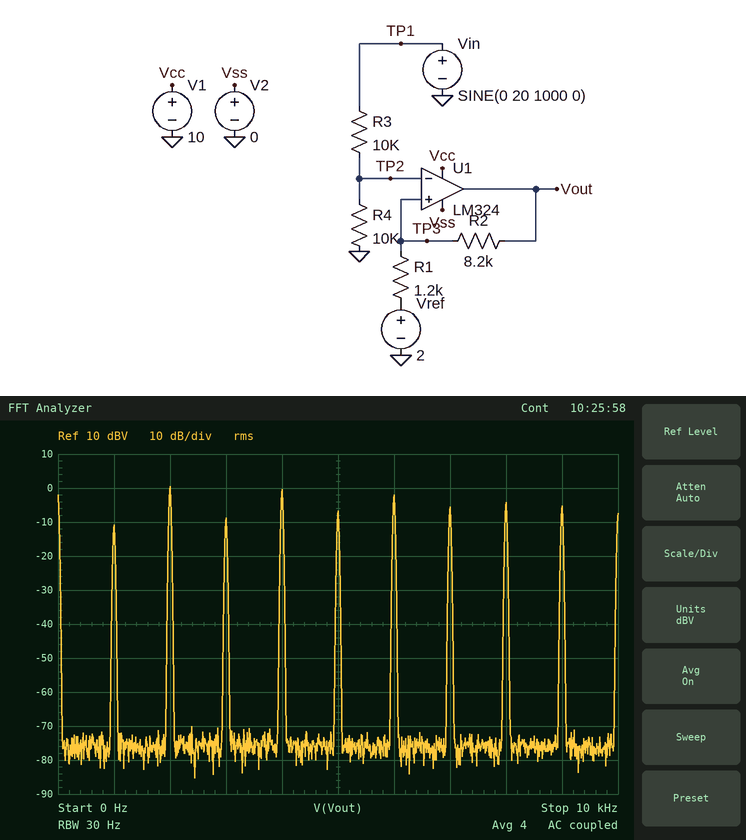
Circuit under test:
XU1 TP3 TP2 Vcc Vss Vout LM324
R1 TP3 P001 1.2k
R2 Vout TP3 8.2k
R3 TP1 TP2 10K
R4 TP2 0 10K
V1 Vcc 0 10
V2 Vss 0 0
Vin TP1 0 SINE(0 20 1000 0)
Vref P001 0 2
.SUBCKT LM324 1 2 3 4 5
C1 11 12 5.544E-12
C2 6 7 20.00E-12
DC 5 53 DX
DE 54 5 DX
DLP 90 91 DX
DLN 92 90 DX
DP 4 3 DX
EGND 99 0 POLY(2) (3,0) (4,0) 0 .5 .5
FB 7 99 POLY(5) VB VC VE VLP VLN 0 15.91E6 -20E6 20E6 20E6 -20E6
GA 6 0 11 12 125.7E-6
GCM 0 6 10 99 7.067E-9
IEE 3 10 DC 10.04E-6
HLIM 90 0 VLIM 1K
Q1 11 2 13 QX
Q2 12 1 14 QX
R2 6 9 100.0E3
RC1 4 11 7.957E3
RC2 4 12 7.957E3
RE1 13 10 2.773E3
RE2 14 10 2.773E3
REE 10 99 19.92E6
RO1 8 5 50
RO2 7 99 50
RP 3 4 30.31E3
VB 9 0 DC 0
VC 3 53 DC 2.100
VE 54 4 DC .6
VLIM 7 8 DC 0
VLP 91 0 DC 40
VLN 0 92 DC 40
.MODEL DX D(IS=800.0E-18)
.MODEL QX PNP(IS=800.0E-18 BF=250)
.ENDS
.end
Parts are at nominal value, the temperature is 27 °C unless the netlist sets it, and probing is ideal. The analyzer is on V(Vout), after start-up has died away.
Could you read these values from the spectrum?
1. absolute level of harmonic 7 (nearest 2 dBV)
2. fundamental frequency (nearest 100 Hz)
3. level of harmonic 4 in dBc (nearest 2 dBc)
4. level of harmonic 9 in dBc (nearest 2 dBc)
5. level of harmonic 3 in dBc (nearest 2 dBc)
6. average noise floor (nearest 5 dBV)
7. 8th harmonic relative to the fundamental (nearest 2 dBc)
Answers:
-6 dBV
1.0 kHz
10 dBc
6 dBc
2 dBc
-75 dBV
6 dBc
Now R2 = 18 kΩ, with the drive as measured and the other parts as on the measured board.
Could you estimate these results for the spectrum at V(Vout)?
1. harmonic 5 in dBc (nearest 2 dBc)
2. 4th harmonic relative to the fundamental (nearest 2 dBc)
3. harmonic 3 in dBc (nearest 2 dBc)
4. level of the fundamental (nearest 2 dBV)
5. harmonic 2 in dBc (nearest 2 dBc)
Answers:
6 dBc
14 dBc
4 dBc
-14 dBV
14 dBc
